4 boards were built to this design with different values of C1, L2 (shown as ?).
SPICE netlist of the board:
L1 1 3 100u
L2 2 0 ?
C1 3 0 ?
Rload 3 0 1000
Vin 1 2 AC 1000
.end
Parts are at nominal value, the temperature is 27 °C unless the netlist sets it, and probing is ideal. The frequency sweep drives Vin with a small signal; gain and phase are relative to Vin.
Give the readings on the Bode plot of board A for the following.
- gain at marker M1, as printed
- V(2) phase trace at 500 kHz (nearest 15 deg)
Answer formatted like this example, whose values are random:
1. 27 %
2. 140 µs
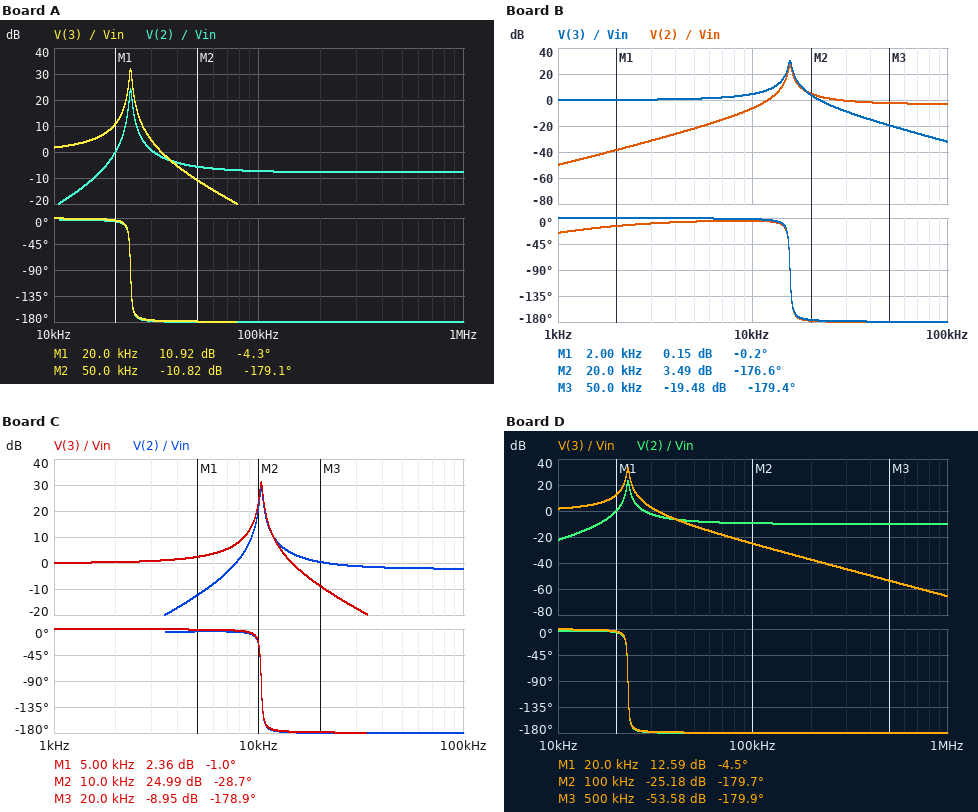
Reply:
1. 10.92 dB
2. -180 deg
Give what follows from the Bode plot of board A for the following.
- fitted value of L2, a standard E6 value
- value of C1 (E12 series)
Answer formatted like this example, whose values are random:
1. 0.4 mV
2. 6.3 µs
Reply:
1. 68 µH
2. 270 nF
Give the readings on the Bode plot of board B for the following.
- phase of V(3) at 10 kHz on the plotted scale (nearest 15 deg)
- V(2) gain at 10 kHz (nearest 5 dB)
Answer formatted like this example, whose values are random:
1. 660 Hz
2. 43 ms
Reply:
1. 0 deg
2. -5 dB
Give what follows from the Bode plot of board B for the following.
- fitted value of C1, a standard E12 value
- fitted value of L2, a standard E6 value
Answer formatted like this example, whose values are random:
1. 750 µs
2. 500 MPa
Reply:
1. 330 nF
2. 220 µH
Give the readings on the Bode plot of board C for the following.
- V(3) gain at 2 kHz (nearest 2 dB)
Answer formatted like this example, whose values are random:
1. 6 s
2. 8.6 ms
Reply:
1. 0 dB
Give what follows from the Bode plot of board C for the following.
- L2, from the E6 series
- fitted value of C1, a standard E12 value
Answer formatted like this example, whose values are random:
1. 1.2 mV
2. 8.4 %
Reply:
1. 330 µH
2. 560 nF
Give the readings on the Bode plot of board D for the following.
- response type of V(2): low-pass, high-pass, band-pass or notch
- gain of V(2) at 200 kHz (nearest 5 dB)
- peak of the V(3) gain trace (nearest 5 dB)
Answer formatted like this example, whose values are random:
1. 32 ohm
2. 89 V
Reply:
1. high-pass
2. -10 dB
3. 35 dB
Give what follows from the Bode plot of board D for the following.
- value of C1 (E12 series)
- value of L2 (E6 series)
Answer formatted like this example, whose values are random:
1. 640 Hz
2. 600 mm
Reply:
1. 330 nF
2. 47 µH
